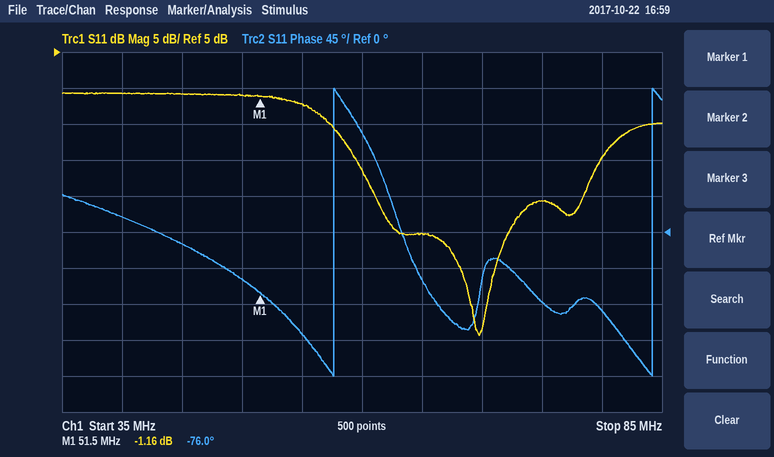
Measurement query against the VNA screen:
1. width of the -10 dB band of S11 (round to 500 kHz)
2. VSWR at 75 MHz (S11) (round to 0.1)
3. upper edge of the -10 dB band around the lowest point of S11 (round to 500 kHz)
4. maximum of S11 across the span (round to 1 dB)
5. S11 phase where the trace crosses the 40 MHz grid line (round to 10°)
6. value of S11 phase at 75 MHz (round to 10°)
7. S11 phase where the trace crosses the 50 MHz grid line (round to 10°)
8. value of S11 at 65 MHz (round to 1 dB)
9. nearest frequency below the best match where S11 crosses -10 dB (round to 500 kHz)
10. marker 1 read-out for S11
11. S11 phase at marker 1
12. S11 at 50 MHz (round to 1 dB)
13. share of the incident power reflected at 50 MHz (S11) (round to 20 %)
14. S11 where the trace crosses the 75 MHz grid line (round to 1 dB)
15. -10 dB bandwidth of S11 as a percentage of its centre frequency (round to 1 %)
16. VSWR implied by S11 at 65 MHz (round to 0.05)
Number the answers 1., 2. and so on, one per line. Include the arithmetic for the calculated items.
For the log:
1. 80.0 MHz − 59.5 MHz = 20.5 MHz
2. |Γ| = 10^(-16/20) = 0.1585; VSWR = (1 + 0.1585)/(1 − 0.1585) ≈ 1.4
3. 80.0 MHz
4. -1 dB
5. 20°
6. -90°
7. -60°
8. -20 dB
9. 59.5 MHz
10. -1.16 dB
11. -76.0°
12. -1 dB
13. 10^(-1/10) ≈ 79.4 %, so 80 % to the nearest 20 %
14. -16 dB
15. 20.5 MHz / 69.75 MHz ≈ 29 %
16. |Γ| = 10^(-20/20) = 0.1000; VSWR = (1 + 0.1000)/(1 − 0.1000) ≈ 1.22, so 1.20 to the nearest 0.05
